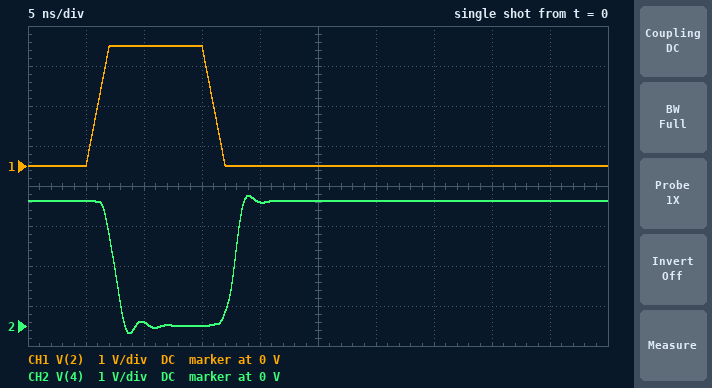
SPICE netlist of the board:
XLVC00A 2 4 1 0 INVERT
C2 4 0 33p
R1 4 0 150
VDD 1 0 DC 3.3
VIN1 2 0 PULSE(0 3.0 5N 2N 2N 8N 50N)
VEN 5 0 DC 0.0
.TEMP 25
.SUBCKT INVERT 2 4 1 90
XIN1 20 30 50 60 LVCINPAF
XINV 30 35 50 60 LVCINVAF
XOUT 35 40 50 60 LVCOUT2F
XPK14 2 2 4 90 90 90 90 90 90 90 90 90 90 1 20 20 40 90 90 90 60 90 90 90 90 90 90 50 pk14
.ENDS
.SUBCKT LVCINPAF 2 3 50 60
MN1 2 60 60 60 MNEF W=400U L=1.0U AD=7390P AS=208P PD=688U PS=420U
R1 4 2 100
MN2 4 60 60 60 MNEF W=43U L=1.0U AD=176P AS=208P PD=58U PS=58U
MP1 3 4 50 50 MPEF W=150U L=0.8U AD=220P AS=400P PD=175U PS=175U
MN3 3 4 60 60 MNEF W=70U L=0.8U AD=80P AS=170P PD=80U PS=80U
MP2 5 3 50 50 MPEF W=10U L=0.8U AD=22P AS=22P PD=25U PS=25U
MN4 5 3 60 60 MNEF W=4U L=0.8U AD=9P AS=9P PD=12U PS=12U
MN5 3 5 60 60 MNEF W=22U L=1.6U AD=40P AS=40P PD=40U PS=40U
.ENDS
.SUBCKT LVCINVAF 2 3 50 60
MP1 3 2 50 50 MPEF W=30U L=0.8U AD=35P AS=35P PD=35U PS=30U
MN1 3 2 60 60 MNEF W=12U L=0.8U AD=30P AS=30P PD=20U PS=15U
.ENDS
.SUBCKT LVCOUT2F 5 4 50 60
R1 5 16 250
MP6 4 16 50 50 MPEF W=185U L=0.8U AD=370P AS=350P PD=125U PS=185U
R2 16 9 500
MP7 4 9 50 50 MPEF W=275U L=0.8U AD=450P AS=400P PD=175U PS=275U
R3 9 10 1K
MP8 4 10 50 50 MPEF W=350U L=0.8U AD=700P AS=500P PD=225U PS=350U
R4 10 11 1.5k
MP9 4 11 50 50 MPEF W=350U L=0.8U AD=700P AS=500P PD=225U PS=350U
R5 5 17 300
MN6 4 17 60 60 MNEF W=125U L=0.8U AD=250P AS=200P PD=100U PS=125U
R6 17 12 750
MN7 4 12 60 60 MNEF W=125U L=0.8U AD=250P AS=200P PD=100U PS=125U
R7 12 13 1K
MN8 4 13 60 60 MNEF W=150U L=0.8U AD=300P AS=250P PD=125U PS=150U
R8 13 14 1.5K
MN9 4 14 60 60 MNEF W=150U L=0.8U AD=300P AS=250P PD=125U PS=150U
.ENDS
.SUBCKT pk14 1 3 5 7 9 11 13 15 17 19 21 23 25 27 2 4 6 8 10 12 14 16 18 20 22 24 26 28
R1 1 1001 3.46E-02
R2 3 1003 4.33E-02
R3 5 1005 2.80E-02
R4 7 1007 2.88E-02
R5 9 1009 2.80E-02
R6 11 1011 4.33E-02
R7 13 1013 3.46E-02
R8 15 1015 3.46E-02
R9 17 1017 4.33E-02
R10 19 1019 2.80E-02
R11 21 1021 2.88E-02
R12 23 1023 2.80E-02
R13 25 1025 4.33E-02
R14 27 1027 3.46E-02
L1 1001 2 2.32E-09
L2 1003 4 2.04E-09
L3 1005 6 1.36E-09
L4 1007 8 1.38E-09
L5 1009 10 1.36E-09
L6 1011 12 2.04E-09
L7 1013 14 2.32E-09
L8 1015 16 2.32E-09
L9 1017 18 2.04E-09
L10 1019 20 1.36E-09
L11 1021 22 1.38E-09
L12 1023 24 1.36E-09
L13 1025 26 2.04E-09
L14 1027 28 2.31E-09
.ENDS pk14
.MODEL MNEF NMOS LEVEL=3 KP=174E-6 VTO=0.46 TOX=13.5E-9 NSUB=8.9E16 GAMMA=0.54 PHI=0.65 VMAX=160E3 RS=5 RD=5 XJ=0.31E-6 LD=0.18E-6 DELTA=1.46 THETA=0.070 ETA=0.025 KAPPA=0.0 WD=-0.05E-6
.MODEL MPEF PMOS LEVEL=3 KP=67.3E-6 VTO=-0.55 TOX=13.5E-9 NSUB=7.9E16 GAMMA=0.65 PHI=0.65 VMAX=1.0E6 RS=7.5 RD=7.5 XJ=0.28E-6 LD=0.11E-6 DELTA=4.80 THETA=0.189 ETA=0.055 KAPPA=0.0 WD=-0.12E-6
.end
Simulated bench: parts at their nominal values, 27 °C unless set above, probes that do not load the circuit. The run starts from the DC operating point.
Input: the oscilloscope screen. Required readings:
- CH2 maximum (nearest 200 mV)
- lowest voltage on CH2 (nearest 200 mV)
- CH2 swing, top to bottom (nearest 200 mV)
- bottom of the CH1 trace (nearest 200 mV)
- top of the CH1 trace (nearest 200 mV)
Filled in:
3.2 V
-200 mV
3.4 V
0 V
3.0 V
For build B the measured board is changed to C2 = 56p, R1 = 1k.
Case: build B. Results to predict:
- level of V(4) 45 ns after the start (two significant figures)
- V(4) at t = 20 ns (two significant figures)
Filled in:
3.3 V
3.4 V
